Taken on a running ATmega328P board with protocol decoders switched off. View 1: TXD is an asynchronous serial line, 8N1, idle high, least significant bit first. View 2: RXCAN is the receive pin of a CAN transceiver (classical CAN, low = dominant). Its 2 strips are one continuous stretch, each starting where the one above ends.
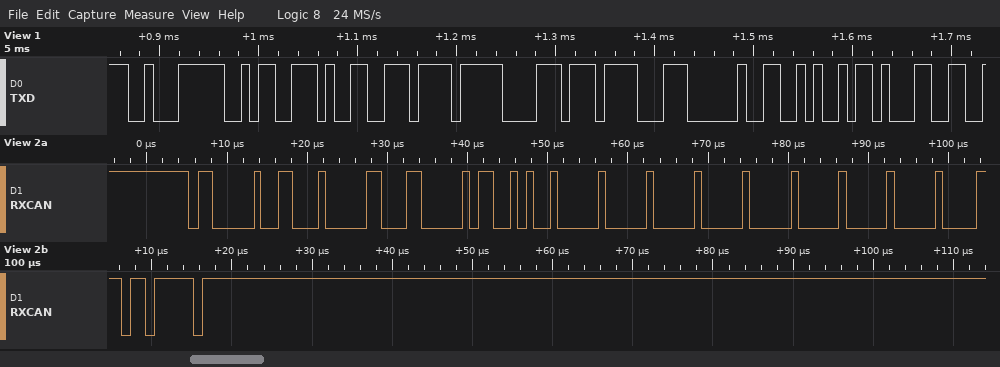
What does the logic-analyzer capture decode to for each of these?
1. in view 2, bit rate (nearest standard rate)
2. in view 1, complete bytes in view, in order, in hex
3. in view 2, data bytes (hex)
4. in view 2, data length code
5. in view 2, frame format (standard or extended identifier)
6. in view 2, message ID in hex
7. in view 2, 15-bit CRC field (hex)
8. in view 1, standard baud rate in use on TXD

1000 kbit/s
E2 9A 99 EF B8 8F 20 4A 31
23 03 29 00 00 00 00 00
8
standard
0x603
0x076F
115200 baud
